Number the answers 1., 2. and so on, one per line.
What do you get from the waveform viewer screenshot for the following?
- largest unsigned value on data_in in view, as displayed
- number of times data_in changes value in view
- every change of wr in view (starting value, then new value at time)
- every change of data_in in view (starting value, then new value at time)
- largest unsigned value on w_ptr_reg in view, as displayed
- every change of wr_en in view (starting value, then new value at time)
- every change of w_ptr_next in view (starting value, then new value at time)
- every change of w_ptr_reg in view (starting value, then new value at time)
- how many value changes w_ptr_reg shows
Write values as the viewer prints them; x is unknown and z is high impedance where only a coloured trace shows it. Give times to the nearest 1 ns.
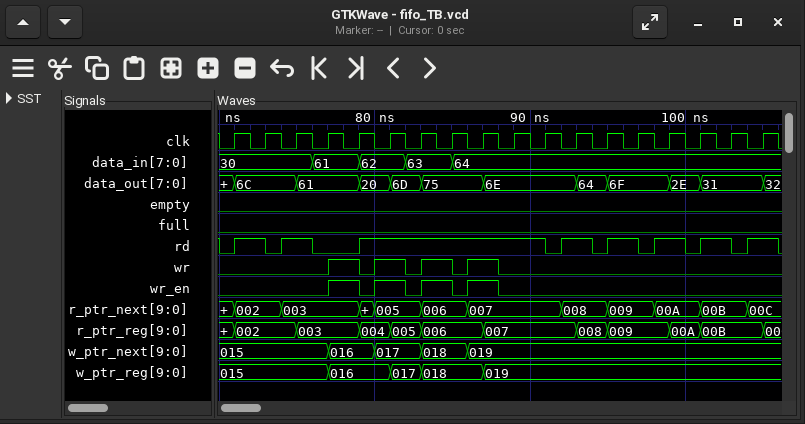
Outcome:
1. 64
2. 4
3. 0, 1 at 77 ns, 0 at 79 ns, 1 at 80 ns, 0 at 82 ns, 1 at 83 ns, 0 at 85 ns, 1 at 86 ns, 0 at 88 ns
4. 30, 61 at 76 ns, 62 at 79 ns, 63 at 82 ns, 64 at 85 ns
5. 019
6. 0, 1 at 77 ns, 0 at 79 ns, 1 at 80 ns, 0 at 82 ns, 1 at 83 ns, 0 at 85 ns, 1 at 86 ns, 0 at 88 ns
7. 015, 016 at 77 ns, 017 at 80 ns, 018 at 83 ns, 019 at 86 ns
8. 015, 016 at 77 ns, 017 at 81 ns, 018 at 83 ns, 019 at 87 ns
9. 4
